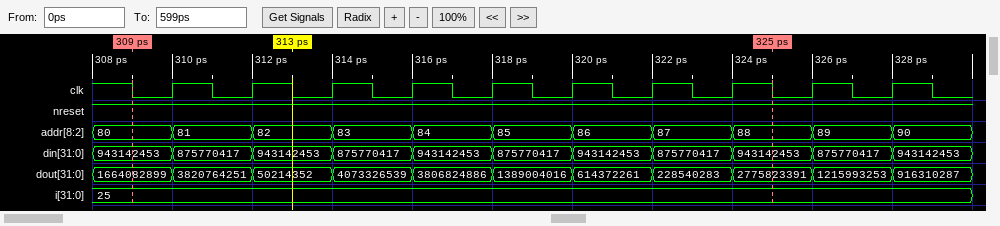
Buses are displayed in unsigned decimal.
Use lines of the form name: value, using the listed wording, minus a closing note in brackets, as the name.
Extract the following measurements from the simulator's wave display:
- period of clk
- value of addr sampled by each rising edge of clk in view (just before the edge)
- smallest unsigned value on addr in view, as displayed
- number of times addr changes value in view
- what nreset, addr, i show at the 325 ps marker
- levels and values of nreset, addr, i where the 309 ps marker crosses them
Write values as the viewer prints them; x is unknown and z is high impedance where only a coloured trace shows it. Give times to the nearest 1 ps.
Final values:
period of clk: 2 ps
value of addr sampled by each rising edge of clk in view: 80, 81, 82, 83, 84, 85, 86, 87, 88, 89
smallest unsigned value on addr in view, as displayed: 80
number of times addr changes value in view: 10
what nreset, addr, i show at the 325 ps marker: nreset=1, addr=88, i=25
levels and values of nreset, addr, i where the 309 ps marker crosses them: nreset=1, addr=80, i=25
